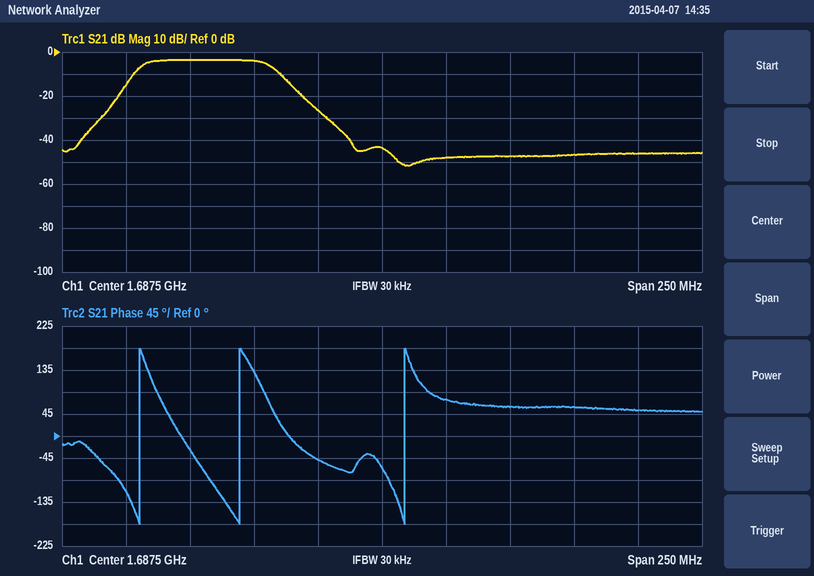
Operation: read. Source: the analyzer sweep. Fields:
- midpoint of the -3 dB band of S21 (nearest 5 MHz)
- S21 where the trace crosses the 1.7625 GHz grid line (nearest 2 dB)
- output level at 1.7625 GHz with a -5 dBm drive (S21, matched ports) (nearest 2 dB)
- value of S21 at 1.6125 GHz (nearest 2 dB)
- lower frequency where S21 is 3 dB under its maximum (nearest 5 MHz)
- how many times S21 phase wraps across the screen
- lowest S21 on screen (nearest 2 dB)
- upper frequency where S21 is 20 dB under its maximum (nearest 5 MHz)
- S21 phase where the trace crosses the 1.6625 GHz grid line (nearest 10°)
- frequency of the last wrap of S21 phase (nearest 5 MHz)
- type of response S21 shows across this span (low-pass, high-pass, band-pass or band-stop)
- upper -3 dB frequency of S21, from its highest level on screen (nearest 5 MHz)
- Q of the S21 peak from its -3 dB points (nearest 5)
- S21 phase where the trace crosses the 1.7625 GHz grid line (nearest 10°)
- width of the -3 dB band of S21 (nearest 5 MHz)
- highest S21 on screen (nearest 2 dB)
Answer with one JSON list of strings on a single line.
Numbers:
["1.620 GHz", "-46 dB", "-52 dBm", "-4 dB", "1.595 GHz", "3", "-52 dB", "1.660 GHz", "-50°", "1.695 GHz", "band-pass", "1.645 GHz", "30", "60°", "50 MHz", "-4 dB"]
